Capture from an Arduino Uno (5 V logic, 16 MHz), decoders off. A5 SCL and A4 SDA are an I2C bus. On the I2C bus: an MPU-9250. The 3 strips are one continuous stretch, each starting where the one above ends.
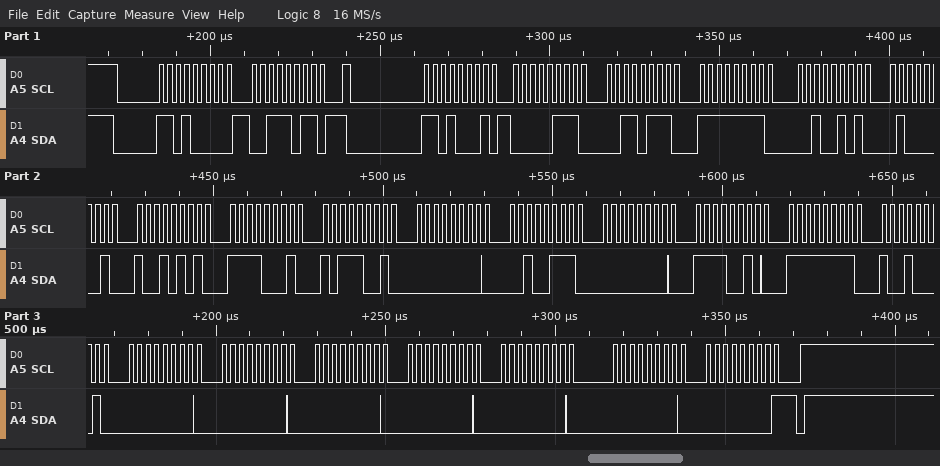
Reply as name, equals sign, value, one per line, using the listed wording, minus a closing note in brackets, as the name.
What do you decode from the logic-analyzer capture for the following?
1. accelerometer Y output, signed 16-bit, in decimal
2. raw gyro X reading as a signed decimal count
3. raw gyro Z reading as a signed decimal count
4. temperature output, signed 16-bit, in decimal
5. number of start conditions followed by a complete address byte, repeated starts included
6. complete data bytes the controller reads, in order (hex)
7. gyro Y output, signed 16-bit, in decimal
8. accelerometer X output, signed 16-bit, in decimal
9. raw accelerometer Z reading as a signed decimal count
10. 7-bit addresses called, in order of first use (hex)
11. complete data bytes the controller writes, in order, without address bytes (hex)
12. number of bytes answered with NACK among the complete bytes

accelerometer Y output, signed 16-bit, in decimal = -219
raw gyro X reading as a signed decimal count = 39
raw gyro Z reading as a signed decimal count = -111
temperature output, signed 16-bit, in decimal = -3655
number of start conditions followed by a complete address byte, repeated starts included = 2
complete data bytes the controller reads, in order = 07 37 FF 25 41 95 F1 B9 00 27 00 F2 FF 91 00 00 00 00 00 00 00
gyro Y output, signed 16-bit, in decimal = 242
accelerometer X output, signed 16-bit, in decimal = 1847
raw accelerometer Z reading as a signed decimal count = 16789
7-bit addresses called, in order of first use = 0x68
complete data bytes the controller writes, in order, without address bytes = 3B
number of bytes answered with NACK among the complete bytes = 1
